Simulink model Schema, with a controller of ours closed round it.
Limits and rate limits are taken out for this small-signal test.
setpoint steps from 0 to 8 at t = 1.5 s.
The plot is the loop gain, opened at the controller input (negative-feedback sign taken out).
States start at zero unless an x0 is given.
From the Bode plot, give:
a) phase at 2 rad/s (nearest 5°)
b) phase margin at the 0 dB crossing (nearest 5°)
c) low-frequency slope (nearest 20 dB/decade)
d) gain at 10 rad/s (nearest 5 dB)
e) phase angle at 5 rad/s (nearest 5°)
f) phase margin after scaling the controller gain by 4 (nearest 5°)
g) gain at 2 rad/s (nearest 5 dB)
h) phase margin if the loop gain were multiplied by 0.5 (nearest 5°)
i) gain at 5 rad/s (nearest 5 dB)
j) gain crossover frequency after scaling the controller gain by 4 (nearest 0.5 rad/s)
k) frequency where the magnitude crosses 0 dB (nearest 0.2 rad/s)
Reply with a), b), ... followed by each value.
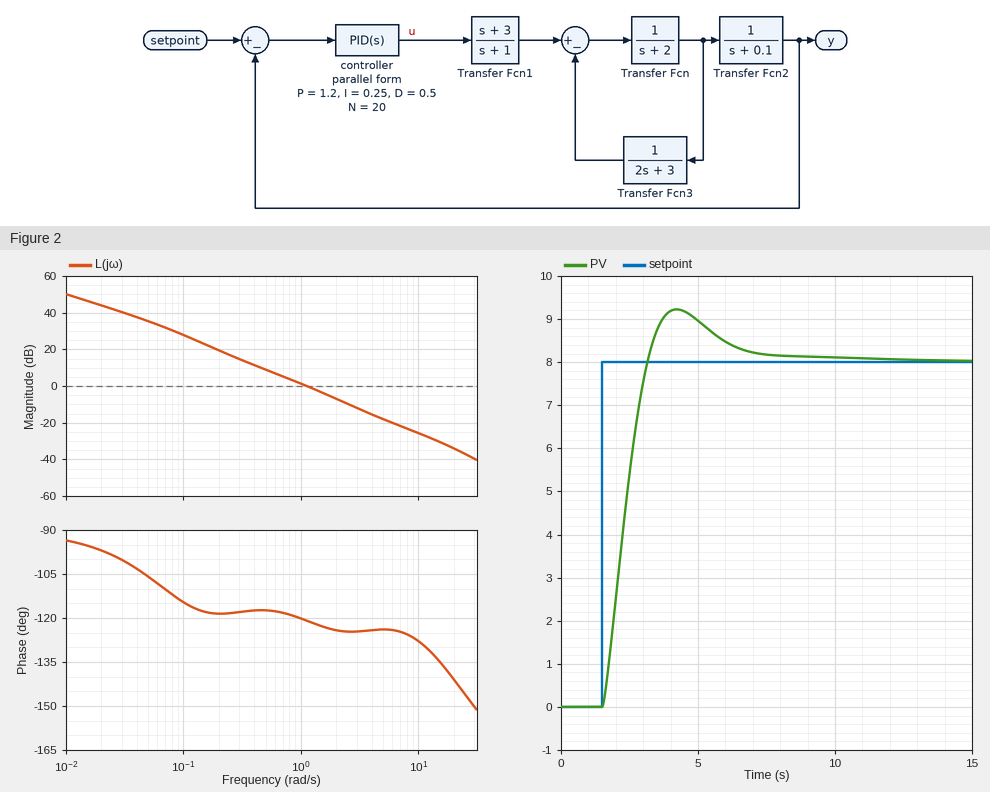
a) -125°
b) 60°
c) -20 dB/decade
d) -25 dB
e) -125°
f) 55°
g) -5 dB
h) 60°
i) -20 dB
j) 3.0 rad/s
k) 1.2 rad/s
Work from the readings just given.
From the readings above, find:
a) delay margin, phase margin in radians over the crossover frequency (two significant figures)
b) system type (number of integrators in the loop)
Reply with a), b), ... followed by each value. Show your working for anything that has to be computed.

a) 60 × π / 180 / 1.2 = 0.87 s
b) 1
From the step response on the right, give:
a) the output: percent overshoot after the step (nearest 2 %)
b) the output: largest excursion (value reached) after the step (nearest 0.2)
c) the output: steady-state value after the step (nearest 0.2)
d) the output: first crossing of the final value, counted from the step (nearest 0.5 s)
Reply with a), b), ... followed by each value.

a) 16 %
b) 9.2
c) 8.0
d) 1.5 s
